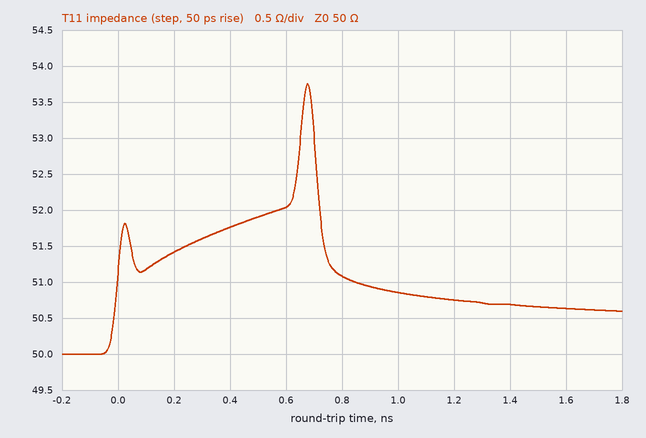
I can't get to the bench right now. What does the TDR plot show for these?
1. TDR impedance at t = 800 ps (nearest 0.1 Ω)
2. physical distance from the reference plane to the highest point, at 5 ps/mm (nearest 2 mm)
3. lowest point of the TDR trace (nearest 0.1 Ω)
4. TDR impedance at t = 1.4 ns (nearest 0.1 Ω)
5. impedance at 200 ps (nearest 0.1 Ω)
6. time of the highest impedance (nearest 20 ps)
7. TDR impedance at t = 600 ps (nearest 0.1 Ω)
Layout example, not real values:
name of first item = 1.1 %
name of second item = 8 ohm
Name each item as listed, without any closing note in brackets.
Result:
TDR impedance at t = 800 ps = 51.1 Ω
physical distance from the reference plane to the highest point, at 5 ps/mm = 68 mm
lowest point of the TDR trace = 50.0 Ω
TDR impedance at t = 1.4 ns = 50.7 Ω
impedance at 200 ps = 51.4 Ω
time of the highest impedance = 680 ps
TDR impedance at t = 600 ps = 52.0 Ω
